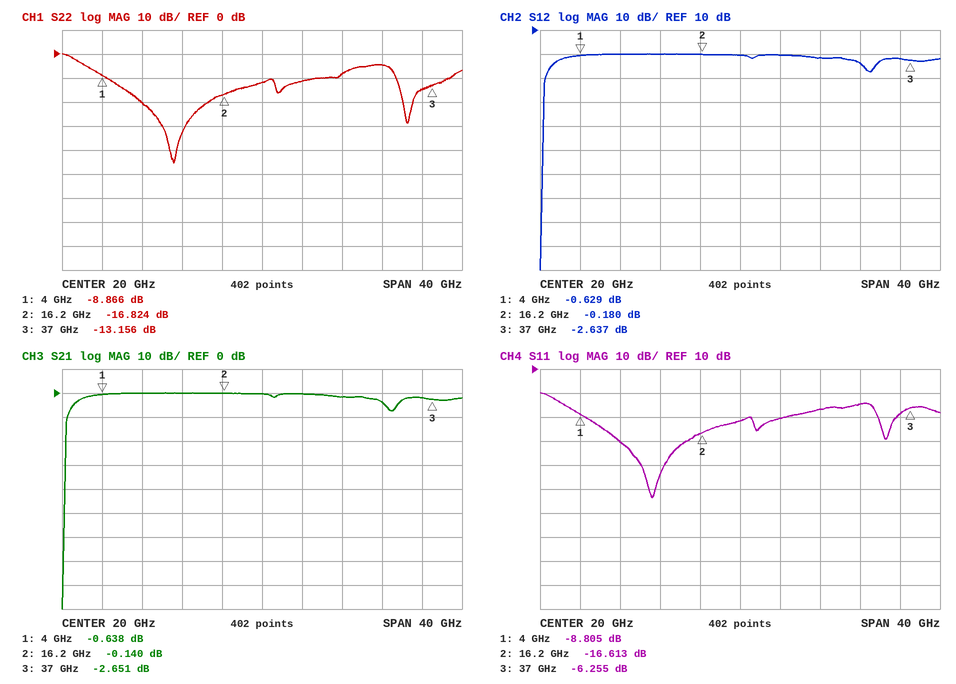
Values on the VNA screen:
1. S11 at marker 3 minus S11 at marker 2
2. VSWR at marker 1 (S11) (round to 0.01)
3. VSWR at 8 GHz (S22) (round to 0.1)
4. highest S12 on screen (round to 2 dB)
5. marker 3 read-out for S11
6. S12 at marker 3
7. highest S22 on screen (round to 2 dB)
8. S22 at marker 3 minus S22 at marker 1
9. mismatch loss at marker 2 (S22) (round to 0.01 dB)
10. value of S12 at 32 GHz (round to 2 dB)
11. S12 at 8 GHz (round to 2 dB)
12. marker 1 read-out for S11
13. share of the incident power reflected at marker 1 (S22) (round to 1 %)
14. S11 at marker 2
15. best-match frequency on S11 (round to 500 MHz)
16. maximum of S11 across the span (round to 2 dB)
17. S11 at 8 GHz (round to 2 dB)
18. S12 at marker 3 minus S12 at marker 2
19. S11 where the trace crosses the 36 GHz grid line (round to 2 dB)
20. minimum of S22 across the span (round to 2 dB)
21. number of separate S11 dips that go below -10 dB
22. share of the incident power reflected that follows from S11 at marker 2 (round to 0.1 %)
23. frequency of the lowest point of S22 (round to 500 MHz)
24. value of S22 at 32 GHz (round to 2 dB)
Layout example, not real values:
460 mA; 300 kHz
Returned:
10.358 dB; 2.14; 1.2; 0 dB; -6.255 dB; -2.637 dB; 0 dB; -4.290 dB; 0.09 dB; -4 dB; 0 dB; -8.805 dB; 13 %; -16.613 dB; 11.0 GHz; 0 dB; -20 dB; -2.457 dB; -8 dB; -46 dB; 3; 2.2 %; 11.0 GHz; -4 dB
